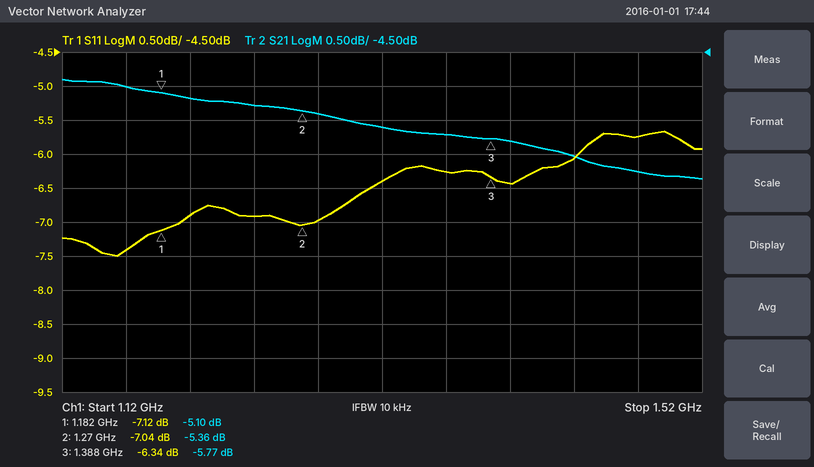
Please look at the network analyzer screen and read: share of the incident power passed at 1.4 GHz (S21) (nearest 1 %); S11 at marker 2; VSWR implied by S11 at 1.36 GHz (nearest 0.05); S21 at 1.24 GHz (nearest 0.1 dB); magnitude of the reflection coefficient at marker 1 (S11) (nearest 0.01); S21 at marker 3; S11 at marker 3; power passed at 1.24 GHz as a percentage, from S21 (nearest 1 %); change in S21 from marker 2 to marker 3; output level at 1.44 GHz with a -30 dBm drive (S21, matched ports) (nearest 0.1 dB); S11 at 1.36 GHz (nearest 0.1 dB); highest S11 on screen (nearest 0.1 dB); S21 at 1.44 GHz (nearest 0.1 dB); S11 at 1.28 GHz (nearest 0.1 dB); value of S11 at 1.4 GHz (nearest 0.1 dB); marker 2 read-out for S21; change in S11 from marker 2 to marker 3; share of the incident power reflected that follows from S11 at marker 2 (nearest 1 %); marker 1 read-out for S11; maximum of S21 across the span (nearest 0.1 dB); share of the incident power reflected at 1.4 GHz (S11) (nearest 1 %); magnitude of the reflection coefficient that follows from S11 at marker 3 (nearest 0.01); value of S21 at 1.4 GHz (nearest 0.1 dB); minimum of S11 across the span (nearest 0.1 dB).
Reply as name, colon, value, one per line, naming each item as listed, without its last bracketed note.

share of the incident power passed at 1.4 GHz (S21): 26 %
S11 at marker 2: -7.04 dB
VSWR implied by S11 at 1.36 GHz: 2.90
S21 at 1.24 GHz: -5.3 dB
magnitude of the reflection coefficient at marker 1 (S11): 0.44
S21 at marker 3: -5.77 dB
S11 at marker 3: -6.34 dB
power passed at 1.24 GHz as a percentage, from S21: 30 %
change in S21 from marker 2 to marker 3: -0.41 dB
output level at 1.44 GHz with a -30 dBm drive (S21, matched ports): -36.0 dBm
S11 at 1.36 GHz: -6.3 dB
highest S11 on screen: -5.7 dB
S21 at 1.44 GHz: -6.0 dB
S11 at 1.28 GHz: -7.0 dB
value of S11 at 1.4 GHz: -6.4 dB
marker 2 read-out for S21: -5.36 dB
change in S11 from marker 2 to marker 3: 0.70 dB
share of the incident power reflected that follows from S11 at marker 2: 20 %
marker 1 read-out for S11: -7.12 dB
maximum of S21 across the span: -4.9 dB
share of the incident power reflected at 1.4 GHz (S11): 23 %
magnitude of the reflection coefficient that follows from S11 at marker 3: 0.48
value of S21 at 1.4 GHz: -5.8 dB
minimum of S11 across the span: -7.5 dB
